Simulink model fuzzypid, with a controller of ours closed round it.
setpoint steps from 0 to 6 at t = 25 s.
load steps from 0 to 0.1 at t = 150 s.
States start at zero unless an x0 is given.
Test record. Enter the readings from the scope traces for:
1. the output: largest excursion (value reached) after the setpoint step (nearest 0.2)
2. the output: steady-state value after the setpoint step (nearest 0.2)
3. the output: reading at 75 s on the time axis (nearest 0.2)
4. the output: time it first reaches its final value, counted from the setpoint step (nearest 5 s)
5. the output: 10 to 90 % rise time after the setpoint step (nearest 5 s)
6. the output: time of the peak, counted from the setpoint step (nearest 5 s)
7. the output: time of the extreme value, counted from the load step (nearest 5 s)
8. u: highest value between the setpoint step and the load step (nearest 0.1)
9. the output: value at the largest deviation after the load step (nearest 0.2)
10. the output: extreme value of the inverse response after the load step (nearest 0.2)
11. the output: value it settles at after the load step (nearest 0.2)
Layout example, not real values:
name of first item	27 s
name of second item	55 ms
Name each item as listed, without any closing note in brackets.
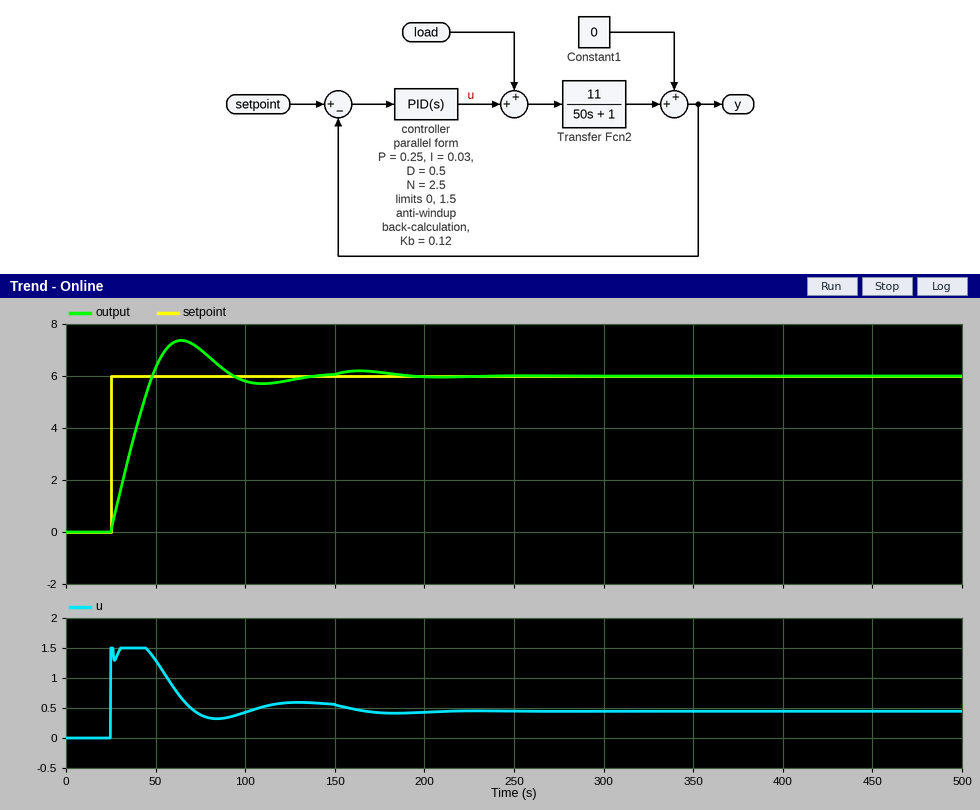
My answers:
the output: largest excursion (value reached) after the setpoint step	7.4
the output: steady-state value after the setpoint step	6.0
the output: reading at 75 s on the time axis	7.0
the output: time it first reaches its final value, counted from the setpoint step	25 s
the output: 10 to 90 % rise time after the setpoint step	20 s
the output: time of the peak, counted from the setpoint step	40 s
the output: time of the extreme value, counted from the load step	60 s
u: highest value between the setpoint step and the load step	1.5
the output: value at the largest deviation after the load step	6.0
the output: extreme value of the inverse response after the load step	6.2
the output: value it settles at after the load step	6.0
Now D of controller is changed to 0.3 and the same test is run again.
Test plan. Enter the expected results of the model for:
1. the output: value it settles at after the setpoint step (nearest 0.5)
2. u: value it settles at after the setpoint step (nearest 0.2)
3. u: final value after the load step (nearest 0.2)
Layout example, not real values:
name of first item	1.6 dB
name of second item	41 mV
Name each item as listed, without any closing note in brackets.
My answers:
the output: value it settles at after the setpoint step	6.0
u: value it settles at after the setpoint step	0.6
u: final value after the load step	0.4
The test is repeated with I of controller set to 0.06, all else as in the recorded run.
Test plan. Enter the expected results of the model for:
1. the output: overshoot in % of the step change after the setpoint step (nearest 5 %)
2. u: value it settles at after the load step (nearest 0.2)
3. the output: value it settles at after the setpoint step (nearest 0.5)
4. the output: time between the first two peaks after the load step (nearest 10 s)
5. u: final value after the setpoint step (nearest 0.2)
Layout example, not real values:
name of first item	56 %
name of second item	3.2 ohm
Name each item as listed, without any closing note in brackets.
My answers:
the output: overshoot in % of the step change after the setpoint step	25 %
u: value it settles at after the load step	0.4
the output: value it settles at after the setpoint step	6.0
the output: time between the first two peaks after the load step	60 s
u: final value after the setpoint step	0.6
